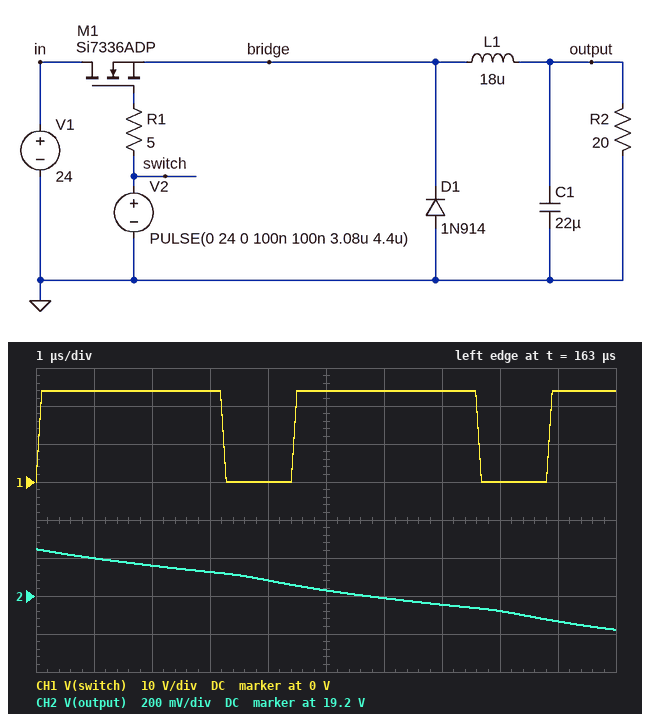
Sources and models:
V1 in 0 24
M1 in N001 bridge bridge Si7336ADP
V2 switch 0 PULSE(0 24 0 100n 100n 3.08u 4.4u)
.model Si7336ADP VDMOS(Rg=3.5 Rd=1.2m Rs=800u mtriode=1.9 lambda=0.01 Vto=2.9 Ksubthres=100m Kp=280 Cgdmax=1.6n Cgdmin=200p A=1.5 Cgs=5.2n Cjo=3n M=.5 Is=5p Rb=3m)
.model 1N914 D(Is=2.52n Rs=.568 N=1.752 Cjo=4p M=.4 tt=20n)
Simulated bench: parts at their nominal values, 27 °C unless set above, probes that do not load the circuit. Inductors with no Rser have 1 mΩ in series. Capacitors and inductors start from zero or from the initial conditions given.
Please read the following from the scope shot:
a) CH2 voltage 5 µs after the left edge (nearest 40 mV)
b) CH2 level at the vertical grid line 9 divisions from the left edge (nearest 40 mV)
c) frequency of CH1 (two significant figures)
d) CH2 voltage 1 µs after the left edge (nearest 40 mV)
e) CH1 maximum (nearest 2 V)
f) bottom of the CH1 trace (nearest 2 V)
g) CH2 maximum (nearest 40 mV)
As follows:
19.24 V
19.08 V
230 kHz
19.40 V
24 V
0 V
19.44 V
